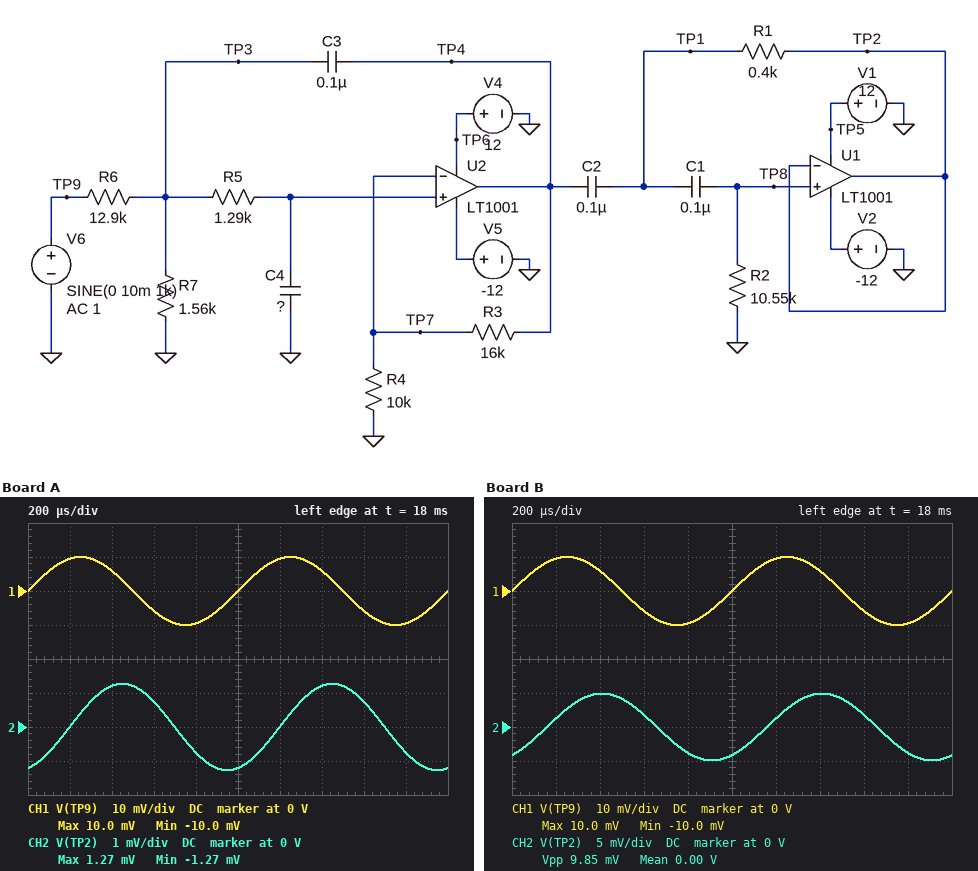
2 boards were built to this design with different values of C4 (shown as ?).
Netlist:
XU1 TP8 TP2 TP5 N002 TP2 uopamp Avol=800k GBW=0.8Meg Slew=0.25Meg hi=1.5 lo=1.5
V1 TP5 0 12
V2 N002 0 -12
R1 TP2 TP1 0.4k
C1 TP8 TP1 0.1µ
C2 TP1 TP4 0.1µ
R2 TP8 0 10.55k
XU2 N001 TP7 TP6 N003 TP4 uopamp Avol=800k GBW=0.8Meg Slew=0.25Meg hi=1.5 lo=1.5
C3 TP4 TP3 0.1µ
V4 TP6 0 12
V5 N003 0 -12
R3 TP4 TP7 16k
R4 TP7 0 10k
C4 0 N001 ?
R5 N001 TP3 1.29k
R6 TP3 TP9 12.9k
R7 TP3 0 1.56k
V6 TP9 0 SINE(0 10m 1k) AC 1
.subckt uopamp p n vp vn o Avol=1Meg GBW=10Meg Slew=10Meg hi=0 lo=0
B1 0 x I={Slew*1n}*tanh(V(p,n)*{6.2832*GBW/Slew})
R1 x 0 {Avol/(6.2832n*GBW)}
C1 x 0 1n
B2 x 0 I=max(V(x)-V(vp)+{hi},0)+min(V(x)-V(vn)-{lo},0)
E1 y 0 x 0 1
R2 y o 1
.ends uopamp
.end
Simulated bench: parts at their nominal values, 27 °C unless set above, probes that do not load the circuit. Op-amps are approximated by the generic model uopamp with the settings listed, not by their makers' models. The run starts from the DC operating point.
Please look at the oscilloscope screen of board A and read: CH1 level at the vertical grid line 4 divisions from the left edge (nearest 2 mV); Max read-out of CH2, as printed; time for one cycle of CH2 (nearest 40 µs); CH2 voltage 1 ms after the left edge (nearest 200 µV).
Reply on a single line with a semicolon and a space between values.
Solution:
-10 mV; 1.27 mV; 1.00 ms; -1.2 mV
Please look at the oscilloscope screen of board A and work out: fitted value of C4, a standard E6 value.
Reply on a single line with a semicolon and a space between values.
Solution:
330 nF
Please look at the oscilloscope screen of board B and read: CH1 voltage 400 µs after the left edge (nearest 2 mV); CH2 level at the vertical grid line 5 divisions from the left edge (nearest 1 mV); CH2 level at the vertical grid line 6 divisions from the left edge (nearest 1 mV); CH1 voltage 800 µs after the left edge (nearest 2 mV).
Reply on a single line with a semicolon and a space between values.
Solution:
6 mV; -4 mV; 1 mV; -10 mV
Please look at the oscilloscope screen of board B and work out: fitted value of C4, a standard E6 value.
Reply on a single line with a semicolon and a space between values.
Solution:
150 nF
